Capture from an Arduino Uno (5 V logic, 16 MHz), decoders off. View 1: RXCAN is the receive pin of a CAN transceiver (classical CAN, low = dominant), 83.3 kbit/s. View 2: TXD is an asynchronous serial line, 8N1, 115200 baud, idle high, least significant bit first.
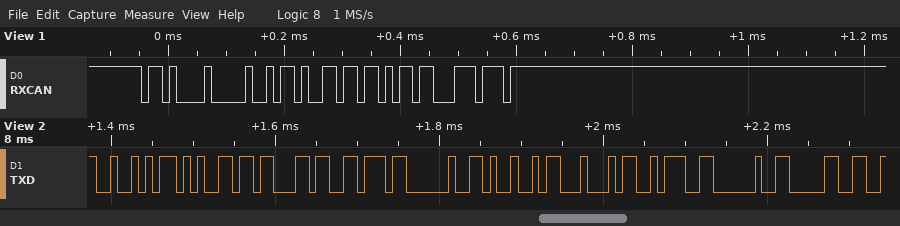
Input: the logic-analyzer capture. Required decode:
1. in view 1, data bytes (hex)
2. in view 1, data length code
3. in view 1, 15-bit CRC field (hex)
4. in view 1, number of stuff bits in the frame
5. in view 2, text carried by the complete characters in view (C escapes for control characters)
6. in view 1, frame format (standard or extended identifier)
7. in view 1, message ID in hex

D3 6D
2
0x363B
1
"Recv ID: 0"
standard
0x684
